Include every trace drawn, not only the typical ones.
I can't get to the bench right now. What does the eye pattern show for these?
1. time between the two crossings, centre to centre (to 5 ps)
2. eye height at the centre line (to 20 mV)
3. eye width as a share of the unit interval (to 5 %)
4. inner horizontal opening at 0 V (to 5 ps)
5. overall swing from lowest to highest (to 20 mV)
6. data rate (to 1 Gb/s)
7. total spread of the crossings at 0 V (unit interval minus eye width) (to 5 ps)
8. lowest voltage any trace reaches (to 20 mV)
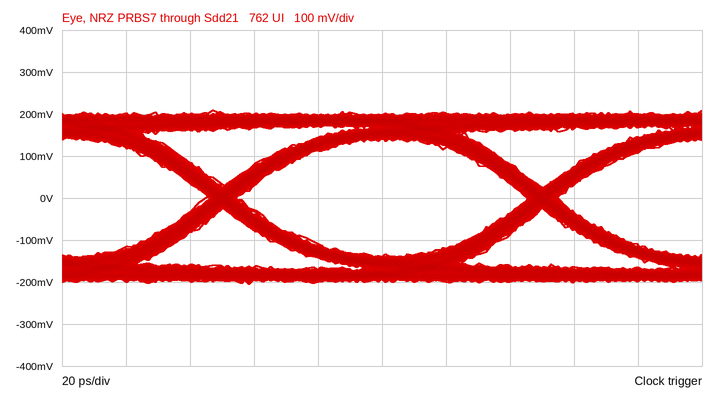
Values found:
100 ps
280 mV
90 %
90 ps
420 mV
10 Gb/s
10 ps
-200 mV
